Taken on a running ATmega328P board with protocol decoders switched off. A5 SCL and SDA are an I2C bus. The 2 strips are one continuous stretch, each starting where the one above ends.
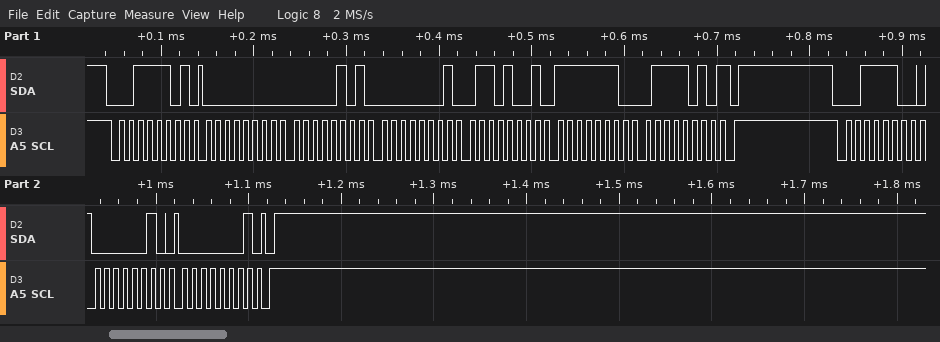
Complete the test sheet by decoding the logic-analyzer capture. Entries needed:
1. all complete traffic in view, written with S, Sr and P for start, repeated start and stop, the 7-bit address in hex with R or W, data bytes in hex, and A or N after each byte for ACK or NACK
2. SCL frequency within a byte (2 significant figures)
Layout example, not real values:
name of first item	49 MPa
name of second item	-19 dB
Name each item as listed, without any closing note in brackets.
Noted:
all complete traffic in view, written with S, Sr and P for start, repeated start and stop, the 7-bit address in hex with R or W, data bytes in hex, and A or N after each byte for ACK or NACK	S 1ER A 00 A 05 A 01 A 69 A FE A 7A N P S 1EW A 02 A 01 A P
SCL frequency within a byte	100 kHz
